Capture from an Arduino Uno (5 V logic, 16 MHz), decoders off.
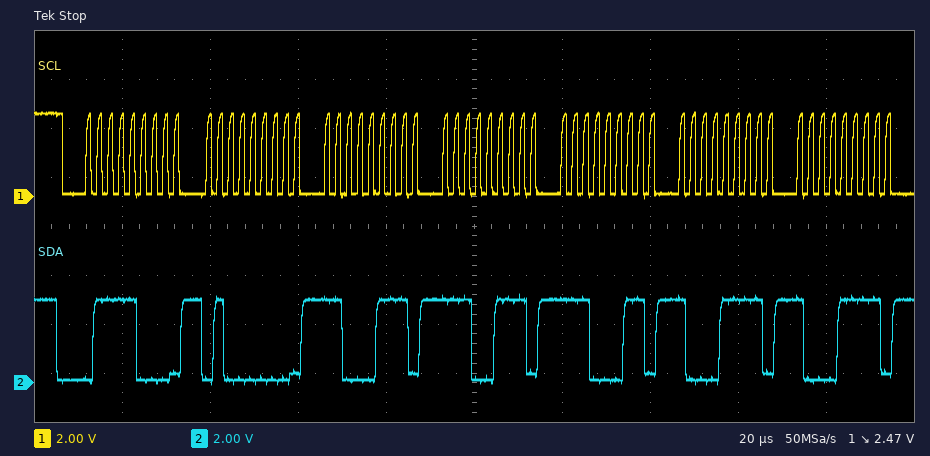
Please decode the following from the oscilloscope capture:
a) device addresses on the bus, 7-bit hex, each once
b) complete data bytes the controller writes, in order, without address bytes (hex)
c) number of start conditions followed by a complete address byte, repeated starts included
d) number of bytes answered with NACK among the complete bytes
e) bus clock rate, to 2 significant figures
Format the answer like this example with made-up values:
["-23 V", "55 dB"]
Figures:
["0x3C", "40 C7 E7 E3 8F 8F", "1", "0", "400 kHz"]
